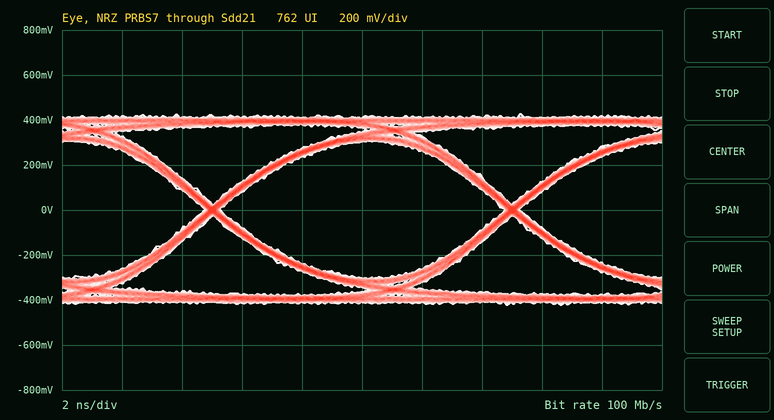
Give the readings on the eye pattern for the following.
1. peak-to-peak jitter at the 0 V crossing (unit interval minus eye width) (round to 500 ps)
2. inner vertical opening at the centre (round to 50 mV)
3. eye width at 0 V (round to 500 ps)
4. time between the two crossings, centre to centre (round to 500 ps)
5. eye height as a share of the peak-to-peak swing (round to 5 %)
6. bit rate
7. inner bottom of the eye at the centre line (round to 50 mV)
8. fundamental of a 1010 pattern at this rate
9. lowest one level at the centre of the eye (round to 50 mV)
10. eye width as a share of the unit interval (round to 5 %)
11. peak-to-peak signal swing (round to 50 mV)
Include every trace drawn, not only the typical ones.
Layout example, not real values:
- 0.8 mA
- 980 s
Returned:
- 500 ps
- 600 mV
- 9.5 ns
- 10.0 ns
- 70 %
- 100 Mb/s
- -300 mV
- 50 MHz
- 300 mV
- 95 %
- 850 mV
